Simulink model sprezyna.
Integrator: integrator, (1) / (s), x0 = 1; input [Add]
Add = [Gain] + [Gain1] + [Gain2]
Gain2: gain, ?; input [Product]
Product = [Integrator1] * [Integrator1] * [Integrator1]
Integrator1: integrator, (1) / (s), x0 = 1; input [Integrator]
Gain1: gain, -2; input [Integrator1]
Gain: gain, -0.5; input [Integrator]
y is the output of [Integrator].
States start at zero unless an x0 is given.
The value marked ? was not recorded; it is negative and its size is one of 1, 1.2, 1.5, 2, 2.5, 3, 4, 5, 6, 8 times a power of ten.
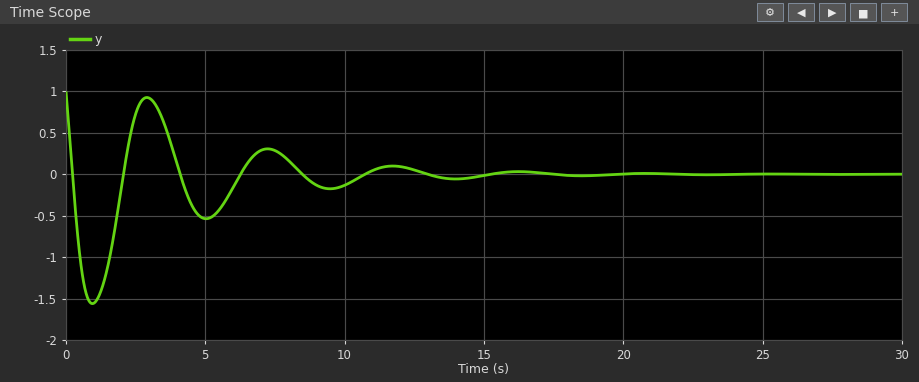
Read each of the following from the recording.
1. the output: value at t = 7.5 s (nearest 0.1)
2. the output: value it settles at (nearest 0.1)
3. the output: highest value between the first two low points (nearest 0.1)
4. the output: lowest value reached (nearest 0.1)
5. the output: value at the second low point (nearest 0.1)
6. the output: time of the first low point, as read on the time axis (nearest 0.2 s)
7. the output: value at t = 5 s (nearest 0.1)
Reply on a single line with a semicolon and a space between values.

0.3; 0.0; 0.9; -1.6; -0.5; 1.0 s; -0.5
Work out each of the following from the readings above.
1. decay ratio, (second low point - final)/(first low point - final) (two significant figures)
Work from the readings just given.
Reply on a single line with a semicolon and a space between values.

0.31
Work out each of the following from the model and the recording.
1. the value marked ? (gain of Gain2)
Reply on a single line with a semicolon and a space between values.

-1.5
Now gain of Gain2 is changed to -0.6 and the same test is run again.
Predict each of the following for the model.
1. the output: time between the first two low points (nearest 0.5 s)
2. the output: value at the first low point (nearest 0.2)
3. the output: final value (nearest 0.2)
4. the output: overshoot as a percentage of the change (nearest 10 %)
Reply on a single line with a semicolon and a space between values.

4.5 s; -1.4; 0.0; 140 %
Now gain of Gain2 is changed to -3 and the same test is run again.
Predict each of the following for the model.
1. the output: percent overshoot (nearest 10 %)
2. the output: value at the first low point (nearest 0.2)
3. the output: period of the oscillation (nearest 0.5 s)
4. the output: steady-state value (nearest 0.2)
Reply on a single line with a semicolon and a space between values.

180 %; -1.8; 3.5 s; 0.0
